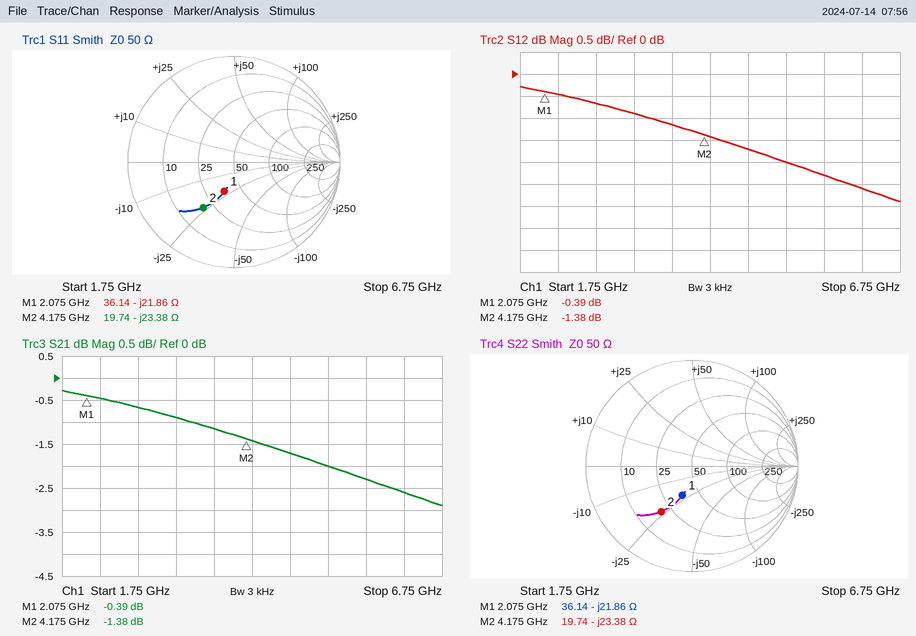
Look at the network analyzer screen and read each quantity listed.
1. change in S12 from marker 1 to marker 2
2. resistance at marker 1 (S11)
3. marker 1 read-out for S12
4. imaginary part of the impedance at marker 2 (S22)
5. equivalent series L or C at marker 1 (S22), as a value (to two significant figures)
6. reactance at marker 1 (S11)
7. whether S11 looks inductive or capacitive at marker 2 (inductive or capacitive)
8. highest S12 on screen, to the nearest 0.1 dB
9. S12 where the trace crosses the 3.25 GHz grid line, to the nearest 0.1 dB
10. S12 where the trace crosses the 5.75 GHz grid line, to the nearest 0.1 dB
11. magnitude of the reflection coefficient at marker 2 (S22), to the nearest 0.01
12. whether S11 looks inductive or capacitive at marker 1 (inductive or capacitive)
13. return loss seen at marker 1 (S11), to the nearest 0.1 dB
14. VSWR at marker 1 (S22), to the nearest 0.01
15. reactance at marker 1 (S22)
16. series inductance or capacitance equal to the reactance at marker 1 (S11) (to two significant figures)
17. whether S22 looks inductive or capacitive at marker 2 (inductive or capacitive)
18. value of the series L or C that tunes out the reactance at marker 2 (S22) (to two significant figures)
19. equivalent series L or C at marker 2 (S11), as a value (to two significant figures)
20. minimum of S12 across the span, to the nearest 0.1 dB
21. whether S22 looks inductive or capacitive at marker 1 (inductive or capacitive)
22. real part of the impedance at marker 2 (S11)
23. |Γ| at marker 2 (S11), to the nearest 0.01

-0.99 dB
36.14 Ω
-0.39 dB
-23.38 Ω
3.5 pF
-21.86 Ω
capacitive
-0.3 dB
-0.9 dB
-2.3 dB
0.52
capacitive
10.7 dB
1.82
-21.86 Ω
3.5 pF
capacitive
890 pH
1.6 pF
-2.9 dB
capacitive
19.74 Ω
0.52
